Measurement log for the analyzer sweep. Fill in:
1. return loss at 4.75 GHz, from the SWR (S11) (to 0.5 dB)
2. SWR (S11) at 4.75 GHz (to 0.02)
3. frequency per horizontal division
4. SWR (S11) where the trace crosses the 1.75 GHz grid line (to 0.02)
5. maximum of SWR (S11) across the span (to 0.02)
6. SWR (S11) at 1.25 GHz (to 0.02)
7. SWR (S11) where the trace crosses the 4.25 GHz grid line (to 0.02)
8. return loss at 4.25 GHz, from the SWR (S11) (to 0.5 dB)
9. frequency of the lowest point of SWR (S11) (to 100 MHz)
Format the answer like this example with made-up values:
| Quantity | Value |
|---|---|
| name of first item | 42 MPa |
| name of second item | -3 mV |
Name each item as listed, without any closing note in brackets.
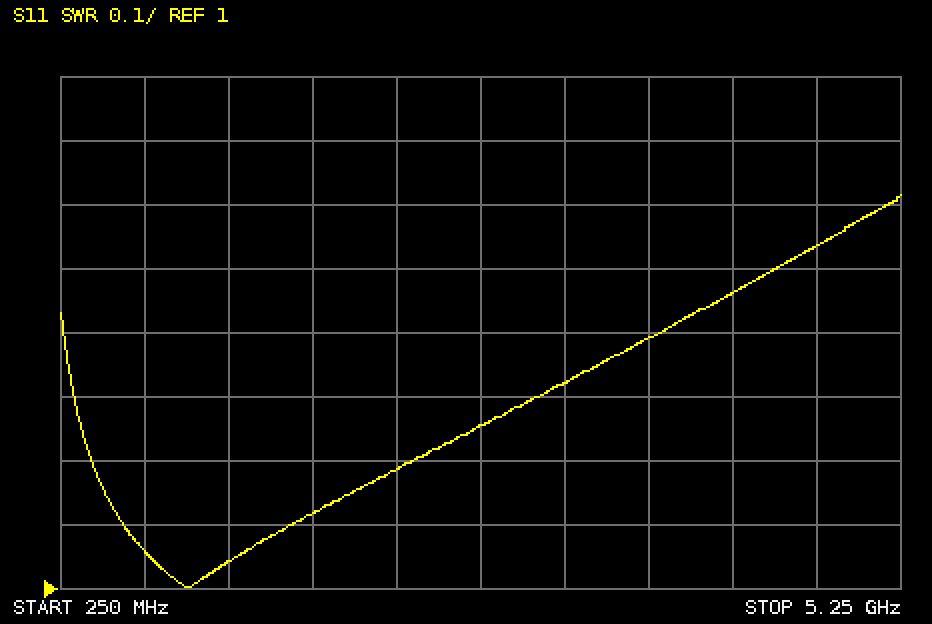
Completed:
| Quantity | Value |
|---|---|
| return loss at 4.75 GHz, from the SWR (S11) | 13.5 dB |
| SWR (S11) at 4.75 GHz | 1.54 |
| frequency per horizontal division | 500 MHz |
| SWR (S11) where the trace crosses the 1.75 GHz grid line | 1.12 |
| maximum of SWR (S11) across the span | 1.62 |
| SWR (S11) at 1.25 GHz | 1.04 |
| SWR (S11) where the trace crosses the 4.25 GHz grid line | 1.46 |
| return loss at 4.25 GHz, from the SWR (S11) | 14.5 dB |
| frequency of the lowest point of SWR (S11) | 1.0 GHz |
